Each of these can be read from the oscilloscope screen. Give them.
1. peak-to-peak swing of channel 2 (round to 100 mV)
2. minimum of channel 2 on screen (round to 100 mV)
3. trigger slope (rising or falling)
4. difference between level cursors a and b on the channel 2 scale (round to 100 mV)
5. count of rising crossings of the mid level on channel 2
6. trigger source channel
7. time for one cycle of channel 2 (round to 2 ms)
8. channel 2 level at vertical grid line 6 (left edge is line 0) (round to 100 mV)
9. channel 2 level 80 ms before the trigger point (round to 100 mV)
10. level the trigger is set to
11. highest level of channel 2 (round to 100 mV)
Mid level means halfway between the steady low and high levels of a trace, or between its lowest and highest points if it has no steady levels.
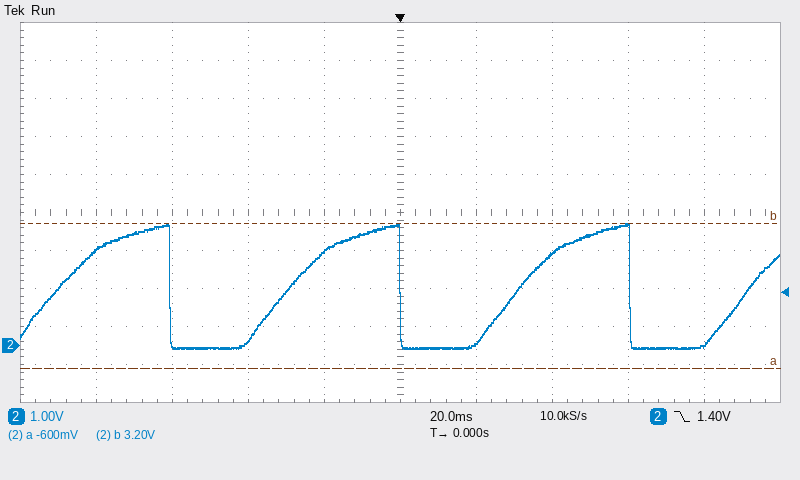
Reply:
3.3 V
-100 mV
falling
3.8 V
4
channel 2
60 ms
100 mV
2.5 V
1.40 V
3.2 V
